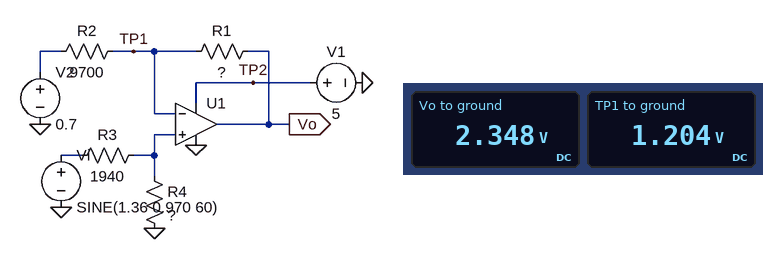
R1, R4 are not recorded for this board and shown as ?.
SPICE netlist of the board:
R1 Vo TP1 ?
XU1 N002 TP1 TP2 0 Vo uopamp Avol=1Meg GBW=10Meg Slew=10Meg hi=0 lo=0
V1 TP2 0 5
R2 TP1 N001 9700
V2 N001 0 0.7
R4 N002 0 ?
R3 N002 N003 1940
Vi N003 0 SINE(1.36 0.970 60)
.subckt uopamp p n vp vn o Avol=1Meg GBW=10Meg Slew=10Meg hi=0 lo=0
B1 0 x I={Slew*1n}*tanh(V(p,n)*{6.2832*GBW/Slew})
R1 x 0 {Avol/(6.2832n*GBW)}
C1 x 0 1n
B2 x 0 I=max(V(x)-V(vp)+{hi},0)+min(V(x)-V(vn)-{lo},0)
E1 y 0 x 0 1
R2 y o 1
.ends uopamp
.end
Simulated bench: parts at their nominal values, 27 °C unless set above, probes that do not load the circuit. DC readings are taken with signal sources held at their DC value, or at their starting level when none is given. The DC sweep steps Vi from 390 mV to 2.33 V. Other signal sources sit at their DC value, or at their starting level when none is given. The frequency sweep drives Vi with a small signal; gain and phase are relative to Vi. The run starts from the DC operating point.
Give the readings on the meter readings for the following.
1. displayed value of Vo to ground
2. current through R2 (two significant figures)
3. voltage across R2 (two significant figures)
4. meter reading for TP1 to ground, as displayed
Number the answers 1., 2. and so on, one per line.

1. 2.348 V
2. 52 µA
3. 500 mV
4. 1.204 V
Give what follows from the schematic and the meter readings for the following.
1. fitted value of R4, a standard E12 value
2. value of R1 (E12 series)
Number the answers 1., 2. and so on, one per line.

1. 15 kΩ
2. 22 kΩ
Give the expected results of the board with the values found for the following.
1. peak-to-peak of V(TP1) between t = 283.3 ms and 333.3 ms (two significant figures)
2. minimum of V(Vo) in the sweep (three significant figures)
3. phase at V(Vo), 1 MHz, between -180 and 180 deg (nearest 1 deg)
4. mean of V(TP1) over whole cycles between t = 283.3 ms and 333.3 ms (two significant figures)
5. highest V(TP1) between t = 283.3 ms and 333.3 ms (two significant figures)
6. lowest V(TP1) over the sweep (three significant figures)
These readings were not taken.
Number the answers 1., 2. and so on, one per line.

1. 1.5 V
2. -6.99 mV
3. -18 deg
4. 1.2 V
5. 2.0 V
6. 484 mV
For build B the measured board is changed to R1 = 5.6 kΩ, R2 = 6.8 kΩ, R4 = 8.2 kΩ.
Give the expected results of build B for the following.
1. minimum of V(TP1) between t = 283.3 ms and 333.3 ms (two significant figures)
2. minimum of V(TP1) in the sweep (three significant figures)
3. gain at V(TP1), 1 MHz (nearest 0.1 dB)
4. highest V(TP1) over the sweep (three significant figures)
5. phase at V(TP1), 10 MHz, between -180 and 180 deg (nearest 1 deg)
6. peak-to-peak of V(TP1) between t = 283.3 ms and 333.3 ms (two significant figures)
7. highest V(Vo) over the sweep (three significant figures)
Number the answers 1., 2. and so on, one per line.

1. 320 mV
2. 316 mV
3. -2.0 dB
4. 1.88 V
5. -61 deg
6. 1.6 V
7. 2.86 V
